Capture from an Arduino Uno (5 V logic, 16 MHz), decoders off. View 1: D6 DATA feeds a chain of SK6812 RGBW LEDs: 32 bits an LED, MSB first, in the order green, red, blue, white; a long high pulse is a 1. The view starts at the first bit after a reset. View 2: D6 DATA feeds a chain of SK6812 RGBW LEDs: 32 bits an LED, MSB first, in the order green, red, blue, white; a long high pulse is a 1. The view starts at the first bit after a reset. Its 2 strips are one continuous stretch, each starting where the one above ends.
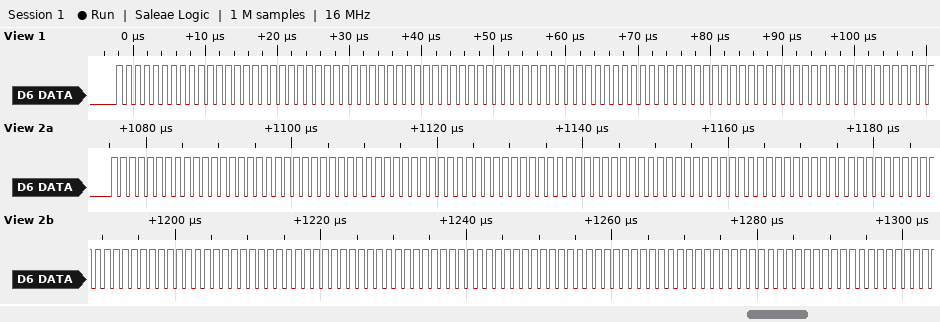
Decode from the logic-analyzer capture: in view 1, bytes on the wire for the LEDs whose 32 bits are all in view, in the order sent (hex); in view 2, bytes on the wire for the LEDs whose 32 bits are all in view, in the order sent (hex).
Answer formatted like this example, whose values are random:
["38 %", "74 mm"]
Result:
["FF FF FF FF FF FF FF FF", "FF FF FF FF FF FF FF FF FF FF FF FF FF FF FF FF FF FF FF FF"]
